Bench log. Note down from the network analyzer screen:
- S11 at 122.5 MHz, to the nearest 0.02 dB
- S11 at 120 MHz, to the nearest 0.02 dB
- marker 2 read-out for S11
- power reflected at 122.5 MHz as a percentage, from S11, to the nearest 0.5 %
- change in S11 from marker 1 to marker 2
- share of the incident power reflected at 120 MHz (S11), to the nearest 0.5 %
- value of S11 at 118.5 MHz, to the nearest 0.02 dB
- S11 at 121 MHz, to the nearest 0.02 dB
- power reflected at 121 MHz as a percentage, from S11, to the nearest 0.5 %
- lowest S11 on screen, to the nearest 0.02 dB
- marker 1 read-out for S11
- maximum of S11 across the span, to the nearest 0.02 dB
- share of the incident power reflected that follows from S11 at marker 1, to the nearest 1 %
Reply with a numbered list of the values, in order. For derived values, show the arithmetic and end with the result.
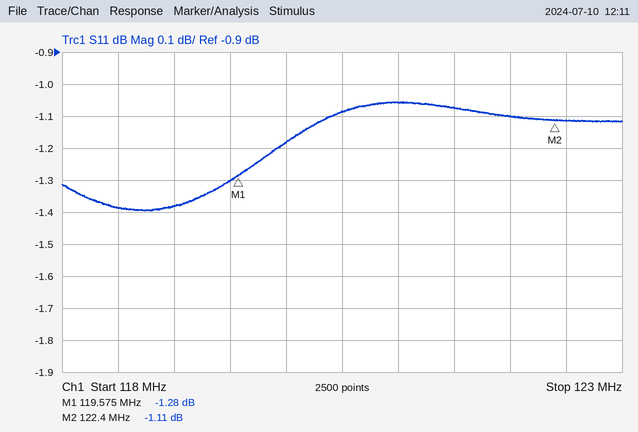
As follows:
1. -1.12 dB
2. -1.18 dB
3. -1.11 dB
4. 10^(-1.12/10) ≈ 77.3 %, so 77.5 % to the nearest 0.5 %
5. -1.11 − (-1.28) = 0.17 dB
6. 10^(-1.18/10) ≈ 76.2 %, so 76.0 % to the nearest 0.5 %
7. -1.38 dB
8. -1.06 dB
9. 10^(-1.06/10) ≈ 78.3 %, so 78.5 % to the nearest 0.5 %
10. -1.40 dB
11. -1.28 dB
12. -1.06 dB
13. 10^(-1.28/10) ≈ 74 %
